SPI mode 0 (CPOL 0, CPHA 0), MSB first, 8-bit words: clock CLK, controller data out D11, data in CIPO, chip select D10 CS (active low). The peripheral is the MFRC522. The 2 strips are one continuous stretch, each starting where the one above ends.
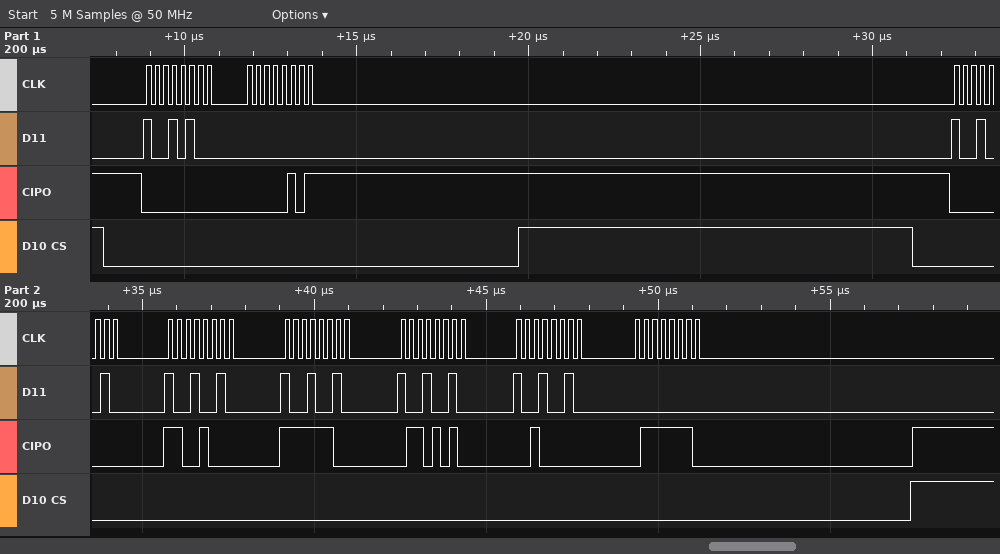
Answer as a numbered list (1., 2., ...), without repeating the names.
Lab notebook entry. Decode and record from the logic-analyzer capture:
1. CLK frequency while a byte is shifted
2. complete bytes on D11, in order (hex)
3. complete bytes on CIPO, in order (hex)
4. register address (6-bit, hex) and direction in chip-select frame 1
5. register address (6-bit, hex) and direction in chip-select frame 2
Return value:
1. 4 MHz
2. 94 00 92 92 92 92 92 00
3. 00 05 00 C8 FC 6A 20 7E
4. 0x0A read
5. 0x09 read
